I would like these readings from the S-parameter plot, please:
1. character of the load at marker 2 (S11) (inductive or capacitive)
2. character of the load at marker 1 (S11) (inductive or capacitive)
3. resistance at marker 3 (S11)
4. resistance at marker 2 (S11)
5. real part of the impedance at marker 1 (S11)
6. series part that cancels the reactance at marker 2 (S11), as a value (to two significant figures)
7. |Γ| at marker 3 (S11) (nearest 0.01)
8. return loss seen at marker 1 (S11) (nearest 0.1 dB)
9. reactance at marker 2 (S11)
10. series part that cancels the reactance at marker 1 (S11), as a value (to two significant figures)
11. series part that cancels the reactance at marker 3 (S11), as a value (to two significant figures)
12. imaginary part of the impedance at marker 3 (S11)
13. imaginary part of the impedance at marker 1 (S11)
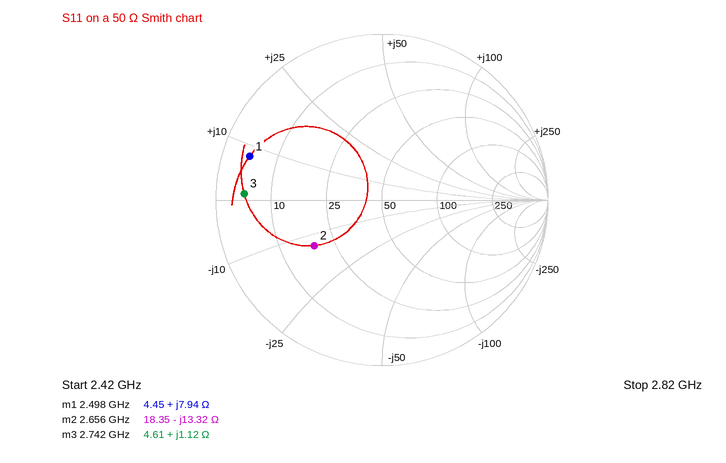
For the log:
capacitive
inductive
4.61 Ω
18.35 Ω
4.45 Ω
800 pH
0.83
1.5 dB
-13.32 Ω
8.0 pF
52 pF
+1.12 Ω
+7.94 Ω
